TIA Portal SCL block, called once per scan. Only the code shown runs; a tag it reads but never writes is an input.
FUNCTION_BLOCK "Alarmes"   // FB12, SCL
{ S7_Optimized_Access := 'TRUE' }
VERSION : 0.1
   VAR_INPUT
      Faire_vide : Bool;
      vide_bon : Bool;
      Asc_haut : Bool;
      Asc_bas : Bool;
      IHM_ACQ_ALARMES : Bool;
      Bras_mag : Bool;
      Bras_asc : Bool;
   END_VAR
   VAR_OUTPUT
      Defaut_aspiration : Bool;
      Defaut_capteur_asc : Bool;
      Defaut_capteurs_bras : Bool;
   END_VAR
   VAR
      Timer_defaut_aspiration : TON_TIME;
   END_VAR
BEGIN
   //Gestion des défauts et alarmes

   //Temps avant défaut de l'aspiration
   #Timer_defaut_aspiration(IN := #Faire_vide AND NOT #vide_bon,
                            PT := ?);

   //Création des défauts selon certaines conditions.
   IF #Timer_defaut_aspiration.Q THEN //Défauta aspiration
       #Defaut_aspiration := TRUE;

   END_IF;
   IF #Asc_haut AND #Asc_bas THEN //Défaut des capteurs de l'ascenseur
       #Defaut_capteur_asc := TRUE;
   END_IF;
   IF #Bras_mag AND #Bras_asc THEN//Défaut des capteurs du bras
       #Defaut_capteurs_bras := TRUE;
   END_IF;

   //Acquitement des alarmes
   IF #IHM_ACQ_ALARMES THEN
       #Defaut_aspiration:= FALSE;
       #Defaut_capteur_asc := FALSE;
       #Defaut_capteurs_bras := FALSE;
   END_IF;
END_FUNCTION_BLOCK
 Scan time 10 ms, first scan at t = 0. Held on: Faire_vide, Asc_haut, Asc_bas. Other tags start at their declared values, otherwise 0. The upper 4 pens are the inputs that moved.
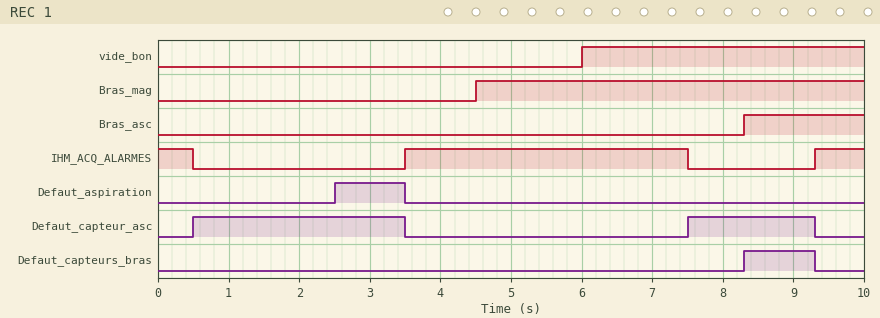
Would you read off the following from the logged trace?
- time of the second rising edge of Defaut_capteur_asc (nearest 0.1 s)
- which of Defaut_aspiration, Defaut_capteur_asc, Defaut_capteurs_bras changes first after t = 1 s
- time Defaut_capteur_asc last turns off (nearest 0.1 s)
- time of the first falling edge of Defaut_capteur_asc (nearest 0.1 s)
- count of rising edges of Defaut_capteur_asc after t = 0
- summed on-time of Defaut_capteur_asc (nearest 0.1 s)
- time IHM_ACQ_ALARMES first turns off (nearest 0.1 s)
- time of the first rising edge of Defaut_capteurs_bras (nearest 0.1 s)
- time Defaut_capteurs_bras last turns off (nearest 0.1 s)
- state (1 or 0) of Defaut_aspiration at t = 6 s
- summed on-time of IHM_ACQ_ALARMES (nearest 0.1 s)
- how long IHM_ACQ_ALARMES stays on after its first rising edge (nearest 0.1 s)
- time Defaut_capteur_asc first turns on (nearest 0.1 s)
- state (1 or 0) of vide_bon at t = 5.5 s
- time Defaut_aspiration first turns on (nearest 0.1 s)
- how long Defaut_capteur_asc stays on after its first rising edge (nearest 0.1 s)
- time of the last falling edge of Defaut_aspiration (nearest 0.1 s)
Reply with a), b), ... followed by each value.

a) 7.5 s
b) Defaut_aspiration
c) 9.3 s
d) 3.5 s
e) 2
f) 4.8 s
g) 0.5 s
h) 8.3 s
i) 9.3 s
j) 0
k) 5.2 s
l) 4.0 s
m) 0.5 s
n) 0
o) 2.5 s
p) 3.0 s
q) 3.5 s
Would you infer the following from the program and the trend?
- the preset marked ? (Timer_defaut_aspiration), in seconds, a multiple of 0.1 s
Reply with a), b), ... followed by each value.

a) 2.5 s
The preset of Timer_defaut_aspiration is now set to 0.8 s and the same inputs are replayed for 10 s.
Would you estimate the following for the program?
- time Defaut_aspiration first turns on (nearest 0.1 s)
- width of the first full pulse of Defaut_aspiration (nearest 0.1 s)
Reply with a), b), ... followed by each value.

a) 0.8 s
b) 2.7 s
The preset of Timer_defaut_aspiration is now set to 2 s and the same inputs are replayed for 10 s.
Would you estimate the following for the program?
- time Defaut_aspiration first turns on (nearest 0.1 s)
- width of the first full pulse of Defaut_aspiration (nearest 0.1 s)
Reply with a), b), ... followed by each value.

a) 2.0 s
b) 1.5 s
